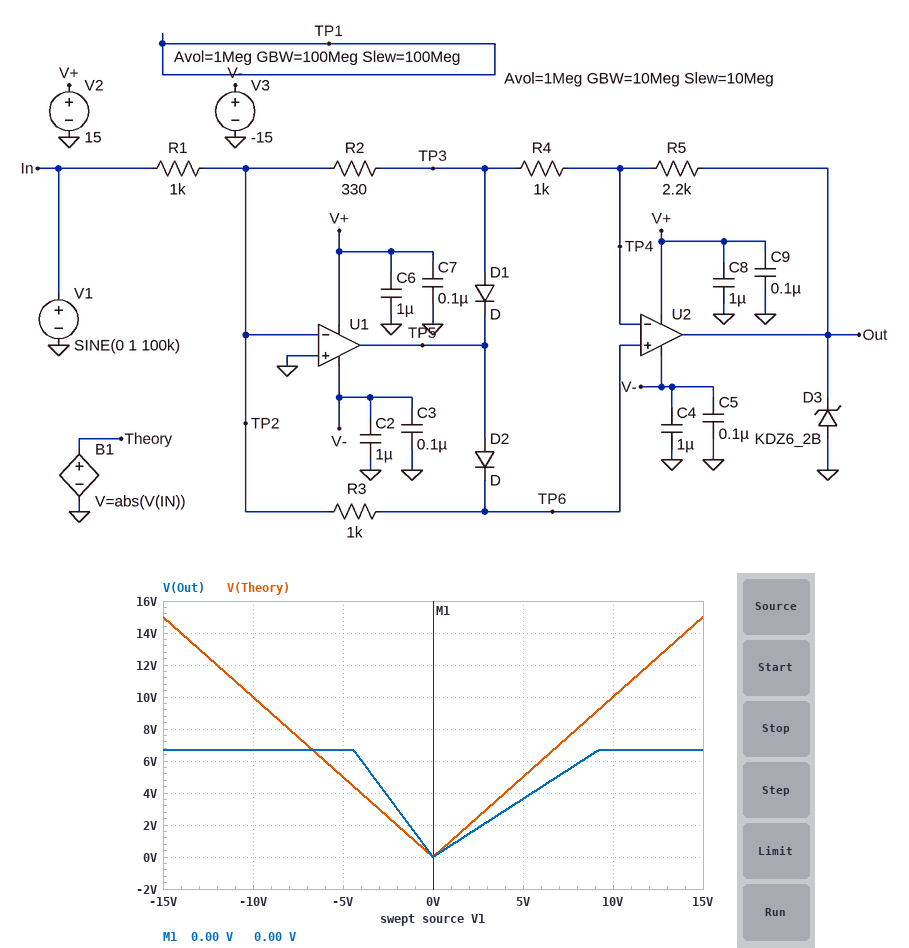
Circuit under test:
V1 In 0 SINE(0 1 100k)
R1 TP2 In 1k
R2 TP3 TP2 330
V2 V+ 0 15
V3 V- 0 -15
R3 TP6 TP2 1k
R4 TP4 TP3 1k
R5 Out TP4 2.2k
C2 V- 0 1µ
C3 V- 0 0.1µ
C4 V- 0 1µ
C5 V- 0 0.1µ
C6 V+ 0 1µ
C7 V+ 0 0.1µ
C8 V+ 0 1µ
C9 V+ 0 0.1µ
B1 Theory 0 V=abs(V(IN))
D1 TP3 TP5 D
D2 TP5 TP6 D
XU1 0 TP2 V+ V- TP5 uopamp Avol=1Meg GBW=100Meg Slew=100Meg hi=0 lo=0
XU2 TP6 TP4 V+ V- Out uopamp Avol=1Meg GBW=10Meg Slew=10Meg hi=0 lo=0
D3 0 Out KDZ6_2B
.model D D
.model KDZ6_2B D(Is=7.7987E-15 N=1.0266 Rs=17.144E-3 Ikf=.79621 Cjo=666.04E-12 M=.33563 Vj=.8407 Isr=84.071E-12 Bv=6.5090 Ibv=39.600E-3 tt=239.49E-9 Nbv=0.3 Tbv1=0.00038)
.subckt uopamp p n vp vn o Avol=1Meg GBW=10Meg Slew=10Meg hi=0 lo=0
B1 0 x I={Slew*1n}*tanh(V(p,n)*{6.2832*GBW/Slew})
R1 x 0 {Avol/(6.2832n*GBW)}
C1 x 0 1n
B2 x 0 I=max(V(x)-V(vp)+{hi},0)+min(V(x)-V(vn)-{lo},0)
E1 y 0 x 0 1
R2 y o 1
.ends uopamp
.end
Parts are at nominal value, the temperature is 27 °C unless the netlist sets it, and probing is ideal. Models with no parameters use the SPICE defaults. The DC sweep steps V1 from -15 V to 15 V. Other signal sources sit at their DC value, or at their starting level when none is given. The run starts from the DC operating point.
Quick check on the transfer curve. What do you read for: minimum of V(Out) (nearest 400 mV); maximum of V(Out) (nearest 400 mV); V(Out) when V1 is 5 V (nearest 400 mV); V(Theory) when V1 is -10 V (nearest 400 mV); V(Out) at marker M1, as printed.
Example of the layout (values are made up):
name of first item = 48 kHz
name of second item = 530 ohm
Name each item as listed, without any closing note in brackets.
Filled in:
minimum of V(Out) = 0 V
maximum of V(Out) = 6.8 V
V(Out) when V1 is 5 V = 3.6 V
V(Theory) when V1 is -10 V = 10.0 V
V(Out) at marker M1, as printed = 0.00 V
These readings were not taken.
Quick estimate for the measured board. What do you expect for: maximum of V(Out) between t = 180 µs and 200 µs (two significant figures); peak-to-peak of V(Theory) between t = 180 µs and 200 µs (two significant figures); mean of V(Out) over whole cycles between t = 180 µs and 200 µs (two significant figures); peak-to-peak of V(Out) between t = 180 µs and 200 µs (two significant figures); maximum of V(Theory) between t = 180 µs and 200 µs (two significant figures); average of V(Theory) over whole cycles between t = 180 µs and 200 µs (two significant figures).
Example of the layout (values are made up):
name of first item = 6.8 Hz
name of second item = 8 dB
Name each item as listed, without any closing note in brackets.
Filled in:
maximum of V(Out) between t = 180 µs and 200 µs = 1.5 V
peak-to-peak of V(Theory) between t = 180 µs and 200 µs = 1.0 V
mean of V(Out) over whole cycles between t = 180 µs and 200 µs = 710 mV
peak-to-peak of V(Out) between t = 180 µs and 200 µs = 1.5 V
maximum of V(Theory) between t = 180 µs and 200 µs = 1.0 V
average of V(Theory) over whole cycles between t = 180 µs and 200 µs = 640 mV
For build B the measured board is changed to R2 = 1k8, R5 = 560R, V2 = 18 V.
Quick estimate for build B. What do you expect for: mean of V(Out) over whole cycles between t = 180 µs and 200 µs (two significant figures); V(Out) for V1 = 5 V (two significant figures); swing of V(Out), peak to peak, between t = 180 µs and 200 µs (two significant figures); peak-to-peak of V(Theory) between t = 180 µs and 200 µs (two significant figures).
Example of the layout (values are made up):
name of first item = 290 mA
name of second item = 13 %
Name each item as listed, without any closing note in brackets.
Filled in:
mean of V(Out) over whole cycles between t = 180 µs and 200 µs = 610 mV
V(Out) for V1 = 5 V = 5.0 V
swing of V(Out), peak to peak, between t = 180 µs and 200 µs = 1.0 V
peak-to-peak of V(Theory) between t = 180 µs and 200 µs = 1.0 V
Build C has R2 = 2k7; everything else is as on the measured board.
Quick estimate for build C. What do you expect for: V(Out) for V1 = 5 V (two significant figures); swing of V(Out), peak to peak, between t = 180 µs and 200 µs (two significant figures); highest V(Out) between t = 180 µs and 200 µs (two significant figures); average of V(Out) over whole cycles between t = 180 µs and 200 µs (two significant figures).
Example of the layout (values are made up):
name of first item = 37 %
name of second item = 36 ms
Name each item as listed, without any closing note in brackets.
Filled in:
V(Out) for V1 = 5 V = 6.7 V
swing of V(Out), peak to peak, between t = 180 µs and 200 µs = 6.0 V
highest V(Out) between t = 180 µs and 200 µs = 5.9 V
average of V(Out) over whole cycles between t = 180 µs and 200 µs = 2.3 V
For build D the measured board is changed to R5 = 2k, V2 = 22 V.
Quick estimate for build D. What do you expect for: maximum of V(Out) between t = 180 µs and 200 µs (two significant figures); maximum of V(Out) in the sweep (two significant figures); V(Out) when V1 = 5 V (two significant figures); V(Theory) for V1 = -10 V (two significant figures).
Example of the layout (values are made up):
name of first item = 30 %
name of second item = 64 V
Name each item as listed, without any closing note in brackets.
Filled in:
maximum of V(Out) between t = 180 µs and 200 µs = 1.4 V
maximum of V(Out) in the sweep = 6.8 V
V(Out) when V1 = 5 V = 3.3 V
V(Theory) for V1 = -10 V = 10 V
